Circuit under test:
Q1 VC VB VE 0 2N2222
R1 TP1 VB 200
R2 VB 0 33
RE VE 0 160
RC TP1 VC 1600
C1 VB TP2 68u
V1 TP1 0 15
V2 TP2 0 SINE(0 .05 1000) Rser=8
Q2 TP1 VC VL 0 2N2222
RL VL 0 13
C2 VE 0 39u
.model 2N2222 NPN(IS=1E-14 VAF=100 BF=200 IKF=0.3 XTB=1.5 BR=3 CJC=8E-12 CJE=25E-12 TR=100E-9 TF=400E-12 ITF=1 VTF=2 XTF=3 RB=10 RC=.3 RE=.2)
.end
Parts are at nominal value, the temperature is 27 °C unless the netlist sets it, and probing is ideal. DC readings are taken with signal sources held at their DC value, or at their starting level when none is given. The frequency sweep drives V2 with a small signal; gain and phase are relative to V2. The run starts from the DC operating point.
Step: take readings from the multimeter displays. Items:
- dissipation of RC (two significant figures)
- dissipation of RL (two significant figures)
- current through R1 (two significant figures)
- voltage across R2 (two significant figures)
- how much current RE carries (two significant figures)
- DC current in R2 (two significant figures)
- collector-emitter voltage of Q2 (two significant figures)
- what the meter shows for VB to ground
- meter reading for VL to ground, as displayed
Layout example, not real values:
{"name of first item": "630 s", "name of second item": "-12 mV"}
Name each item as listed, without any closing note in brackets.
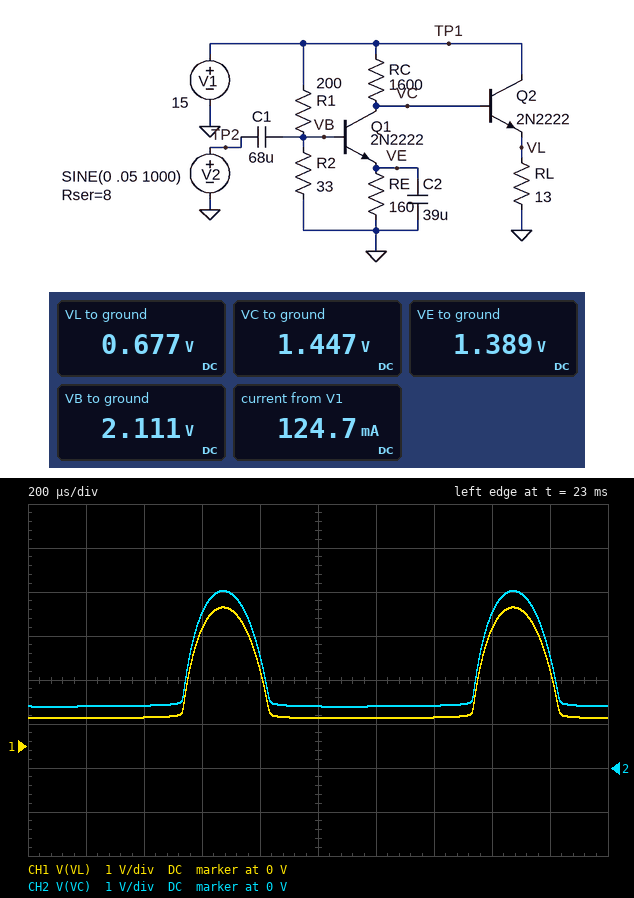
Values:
{"dissipation of RC": "110 mW", "dissipation of RL": "35 mW", "current through R1": "64 mA", "voltage across R2": "2.1 V", "how much current RE carries": "8.7 mA", "DC current in R2": "64 mA", "collector-emitter voltage of Q2": "14 V", "what the meter shows for VB to ground": "2.111 V", "meter reading for VL to ground, as displayed": "0.677 V"}
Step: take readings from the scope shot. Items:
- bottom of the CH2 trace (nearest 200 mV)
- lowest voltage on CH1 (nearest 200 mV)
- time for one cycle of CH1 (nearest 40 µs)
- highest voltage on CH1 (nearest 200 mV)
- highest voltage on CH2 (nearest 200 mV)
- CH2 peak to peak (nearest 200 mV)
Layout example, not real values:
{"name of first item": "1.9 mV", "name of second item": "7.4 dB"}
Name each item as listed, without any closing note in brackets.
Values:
{"bottom of the CH2 trace": "1.4 V", "lowest voltage on CH1": "600 mV", "time for one cycle of CH1": "1.00 ms", "highest voltage on CH1": "3.2 V", "highest voltage on CH2": "4.0 V", "CH2 peak to peak": "2.6 V"}
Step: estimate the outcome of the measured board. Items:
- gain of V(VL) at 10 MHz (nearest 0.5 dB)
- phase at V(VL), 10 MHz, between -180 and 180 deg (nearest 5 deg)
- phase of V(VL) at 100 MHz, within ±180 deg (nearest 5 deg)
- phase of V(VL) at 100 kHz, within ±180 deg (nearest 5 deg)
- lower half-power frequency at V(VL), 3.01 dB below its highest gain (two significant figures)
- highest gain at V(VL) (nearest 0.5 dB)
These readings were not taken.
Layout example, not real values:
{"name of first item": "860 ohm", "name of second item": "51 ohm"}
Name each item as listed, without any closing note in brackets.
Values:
{"gain of V(VL) at 10 MHz": "-16.5 dB", "phase at V(VL), 10 MHz, between -180 and 180 deg": "45 deg", "phase of V(VL) at 100 MHz, within ±180 deg": "-20 deg", "phase of V(VL) at 100 kHz, within ±180 deg": "170 deg", "lower half-power frequency at V(VL), 3.01 dB below its highest gain": "250 Hz", "highest gain at V(VL)": "2.5 dB"}
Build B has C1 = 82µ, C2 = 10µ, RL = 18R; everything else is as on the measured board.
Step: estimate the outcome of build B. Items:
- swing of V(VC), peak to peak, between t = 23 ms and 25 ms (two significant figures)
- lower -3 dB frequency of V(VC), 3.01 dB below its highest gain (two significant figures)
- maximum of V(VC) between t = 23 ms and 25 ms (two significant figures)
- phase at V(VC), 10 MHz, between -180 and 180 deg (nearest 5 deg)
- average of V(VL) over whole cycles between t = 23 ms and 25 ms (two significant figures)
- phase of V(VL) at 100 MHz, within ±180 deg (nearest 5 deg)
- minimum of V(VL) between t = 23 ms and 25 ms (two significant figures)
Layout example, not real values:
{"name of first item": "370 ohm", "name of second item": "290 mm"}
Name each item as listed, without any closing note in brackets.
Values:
{"swing of V(VC), peak to peak, between t = 23 ms and 25 ms": "1.8 V", "lower -3 dB frequency of V(VC), 3.01 dB below its highest gain": "730 Hz", "maximum of V(VC) between t = 23 ms and 25 ms": "3.2 V", "phase at V(VC), 10 MHz, between -180 and 180 deg": "50 deg", "average of V(VL) over whole cycles between t = 23 ms and 25 ms": "1.0 V", "phase of V(VL) at 100 MHz, within ±180 deg": "-15 deg", "minimum of V(VL) between t = 23 ms and 25 ms": "650 mV"}
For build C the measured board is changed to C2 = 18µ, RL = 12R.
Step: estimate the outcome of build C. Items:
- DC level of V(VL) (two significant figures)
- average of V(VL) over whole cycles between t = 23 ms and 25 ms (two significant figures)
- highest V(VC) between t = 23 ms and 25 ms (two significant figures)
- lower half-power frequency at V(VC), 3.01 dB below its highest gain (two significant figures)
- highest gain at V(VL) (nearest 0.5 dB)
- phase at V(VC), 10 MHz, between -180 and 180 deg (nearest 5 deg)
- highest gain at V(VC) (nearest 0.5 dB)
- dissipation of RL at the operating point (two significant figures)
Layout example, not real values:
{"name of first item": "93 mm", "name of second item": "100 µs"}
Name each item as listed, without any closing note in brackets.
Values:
{"DC level of V(VL)": "670 mV", "average of V(VL) over whole cycles between t = 23 ms and 25 ms": "1.0 V", "highest V(VC) between t = 23 ms and 25 ms": "3.4 V", "lower half-power frequency at V(VC), 3.01 dB below its highest gain": "430 Hz", "highest gain at V(VL)": "2.0 dB", "phase at V(VC), 10 MHz, between -180 and 180 deg": "45 deg", "highest gain at V(VC)": "2.5 dB", "dissipation of RL at the operating point": "38 mW"}
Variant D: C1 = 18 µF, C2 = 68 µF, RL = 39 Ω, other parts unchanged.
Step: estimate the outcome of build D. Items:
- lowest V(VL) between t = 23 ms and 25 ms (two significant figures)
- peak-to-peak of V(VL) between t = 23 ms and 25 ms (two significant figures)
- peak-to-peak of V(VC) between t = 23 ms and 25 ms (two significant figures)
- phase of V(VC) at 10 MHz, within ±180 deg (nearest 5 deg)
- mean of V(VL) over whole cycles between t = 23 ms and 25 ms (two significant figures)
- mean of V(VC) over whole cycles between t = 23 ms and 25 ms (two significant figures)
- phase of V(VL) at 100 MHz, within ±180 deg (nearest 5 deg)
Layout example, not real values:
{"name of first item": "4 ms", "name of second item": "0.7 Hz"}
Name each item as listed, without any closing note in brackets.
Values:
{"lowest V(VL) between t = 23 ms and 25 ms": "670 mV", "peak-to-peak of V(VL) between t = 23 ms and 25 ms": "4.2 V", "peak-to-peak of V(VC) between t = 23 ms and 25 ms": "4.3 V", "phase of V(VC) at 10 MHz, within ±180 deg": "55 deg", "mean of V(VL) over whole cycles between t = 23 ms and 25 ms": "1.6 V", "mean of V(VC) over whole cycles between t = 23 ms and 25 ms": "2.4 V", "phase of V(VL) at 100 MHz, within ±180 deg": "-10 deg"}
